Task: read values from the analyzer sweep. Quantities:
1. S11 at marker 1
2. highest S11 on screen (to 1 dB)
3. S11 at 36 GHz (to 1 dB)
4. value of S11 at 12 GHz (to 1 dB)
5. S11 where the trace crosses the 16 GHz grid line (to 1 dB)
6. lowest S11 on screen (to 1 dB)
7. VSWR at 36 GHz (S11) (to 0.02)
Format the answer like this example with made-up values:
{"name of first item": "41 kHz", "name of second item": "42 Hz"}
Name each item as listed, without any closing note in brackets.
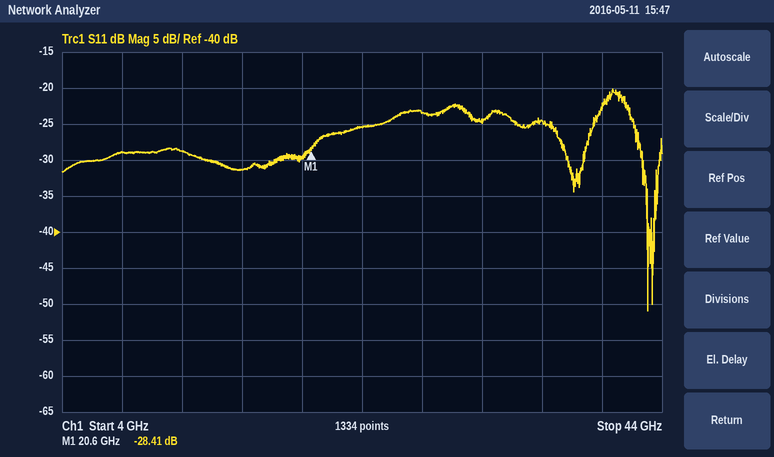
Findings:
{"S11 at marker 1": "-28.41 dB", "highest S11 on screen": "-20 dB", "S11 at 36 GHz": "-25 dB", "value of S11 at 12 GHz": "-29 dB", "S11 where the trace crosses the 16 GHz grid line": "-31 dB", "lowest S11 on screen": "-51 dB", "VSWR at 36 GHz (S11)": "1.12"}
